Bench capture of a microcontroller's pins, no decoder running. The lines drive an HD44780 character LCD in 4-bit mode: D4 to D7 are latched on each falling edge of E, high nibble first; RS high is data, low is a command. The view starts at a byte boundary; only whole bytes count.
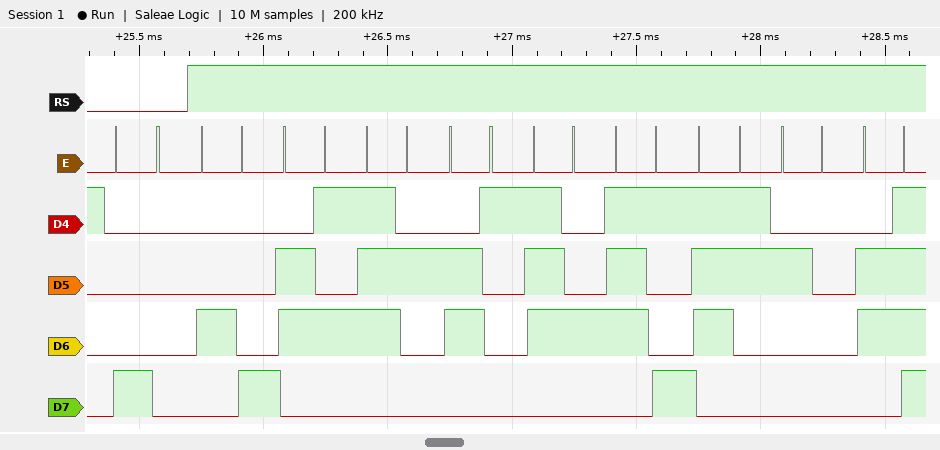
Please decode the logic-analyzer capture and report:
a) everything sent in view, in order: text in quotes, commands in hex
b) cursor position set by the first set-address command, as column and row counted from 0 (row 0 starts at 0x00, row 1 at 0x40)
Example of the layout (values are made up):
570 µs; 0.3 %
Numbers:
0x80 "Heratys o"; column 0, row 0
